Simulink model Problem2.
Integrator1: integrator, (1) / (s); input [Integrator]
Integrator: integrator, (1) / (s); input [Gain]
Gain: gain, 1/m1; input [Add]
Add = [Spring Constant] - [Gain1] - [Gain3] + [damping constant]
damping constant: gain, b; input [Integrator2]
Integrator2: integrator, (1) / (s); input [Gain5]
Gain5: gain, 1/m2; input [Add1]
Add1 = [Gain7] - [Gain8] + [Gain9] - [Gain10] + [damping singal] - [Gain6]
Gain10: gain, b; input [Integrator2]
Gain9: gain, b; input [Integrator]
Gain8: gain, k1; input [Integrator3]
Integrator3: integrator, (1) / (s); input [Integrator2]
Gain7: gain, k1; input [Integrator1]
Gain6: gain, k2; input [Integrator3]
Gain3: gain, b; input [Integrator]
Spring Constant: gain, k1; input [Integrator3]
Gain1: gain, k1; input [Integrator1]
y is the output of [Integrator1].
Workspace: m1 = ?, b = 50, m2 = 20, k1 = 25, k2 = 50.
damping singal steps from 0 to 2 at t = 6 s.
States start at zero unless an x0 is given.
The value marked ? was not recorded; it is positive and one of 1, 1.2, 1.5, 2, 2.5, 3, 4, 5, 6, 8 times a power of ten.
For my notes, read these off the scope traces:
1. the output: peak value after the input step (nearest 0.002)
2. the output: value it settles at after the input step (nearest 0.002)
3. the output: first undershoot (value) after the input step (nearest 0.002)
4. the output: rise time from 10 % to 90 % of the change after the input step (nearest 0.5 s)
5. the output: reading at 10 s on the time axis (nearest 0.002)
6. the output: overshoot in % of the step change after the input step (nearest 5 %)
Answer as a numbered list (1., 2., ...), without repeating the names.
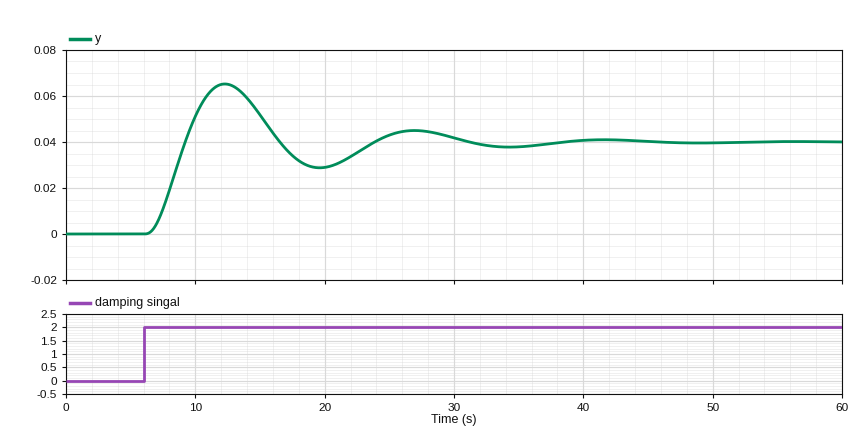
1. 0.066
2. 0.040
3. 0.028
4. 2.0 s
5. 0.052
6. 65 %
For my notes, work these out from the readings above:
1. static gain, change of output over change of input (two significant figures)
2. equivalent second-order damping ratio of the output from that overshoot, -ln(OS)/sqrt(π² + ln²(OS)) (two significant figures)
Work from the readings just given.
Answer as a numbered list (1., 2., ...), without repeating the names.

1. 0.020
2. 0.14
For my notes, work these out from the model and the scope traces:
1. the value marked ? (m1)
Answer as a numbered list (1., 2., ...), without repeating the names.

1. 100
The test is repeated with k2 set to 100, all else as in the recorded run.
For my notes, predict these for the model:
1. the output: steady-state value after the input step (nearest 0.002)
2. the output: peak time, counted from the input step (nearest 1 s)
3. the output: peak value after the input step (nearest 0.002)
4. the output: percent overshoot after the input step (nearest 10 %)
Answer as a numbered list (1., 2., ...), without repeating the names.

1. 0.020
2. 5 s
3. 0.030
4. 50 %
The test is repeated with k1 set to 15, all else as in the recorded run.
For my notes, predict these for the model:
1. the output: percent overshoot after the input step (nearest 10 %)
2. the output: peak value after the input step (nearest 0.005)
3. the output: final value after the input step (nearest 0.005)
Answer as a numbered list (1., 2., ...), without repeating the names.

1. 50 %
2. 0.060
3. 0.040
